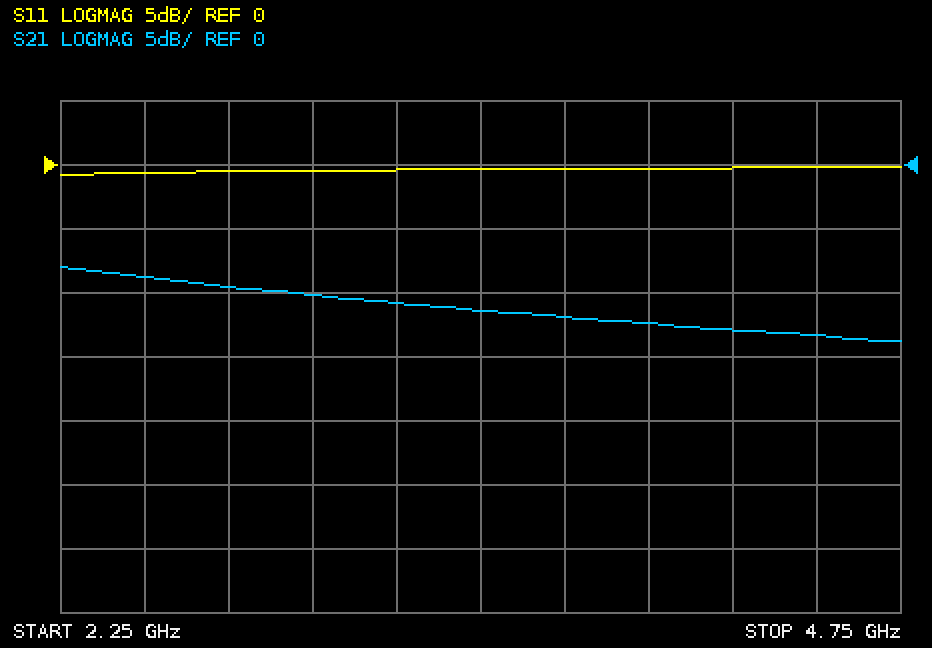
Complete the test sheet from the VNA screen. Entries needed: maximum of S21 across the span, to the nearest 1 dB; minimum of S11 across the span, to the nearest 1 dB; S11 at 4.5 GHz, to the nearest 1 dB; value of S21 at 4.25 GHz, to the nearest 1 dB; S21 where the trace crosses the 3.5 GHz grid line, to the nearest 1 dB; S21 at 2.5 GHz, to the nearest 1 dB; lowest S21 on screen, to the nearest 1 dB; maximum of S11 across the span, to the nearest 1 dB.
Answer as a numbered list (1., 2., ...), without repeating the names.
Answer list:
1. -8 dB
2. -1 dB
3. 0 dB
4. -13 dB
5. -11 dB
6. -9 dB
7. -14 dB
8. 0 dB
